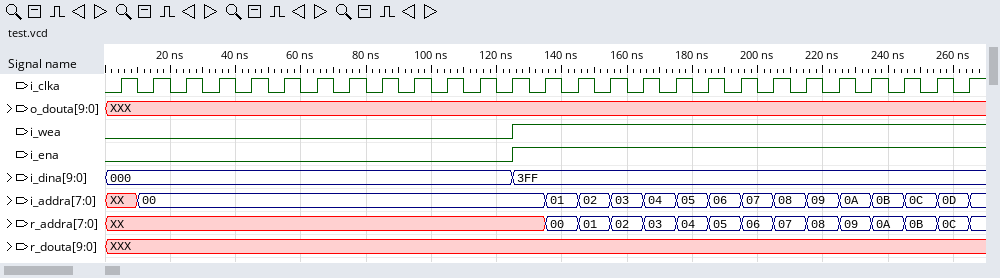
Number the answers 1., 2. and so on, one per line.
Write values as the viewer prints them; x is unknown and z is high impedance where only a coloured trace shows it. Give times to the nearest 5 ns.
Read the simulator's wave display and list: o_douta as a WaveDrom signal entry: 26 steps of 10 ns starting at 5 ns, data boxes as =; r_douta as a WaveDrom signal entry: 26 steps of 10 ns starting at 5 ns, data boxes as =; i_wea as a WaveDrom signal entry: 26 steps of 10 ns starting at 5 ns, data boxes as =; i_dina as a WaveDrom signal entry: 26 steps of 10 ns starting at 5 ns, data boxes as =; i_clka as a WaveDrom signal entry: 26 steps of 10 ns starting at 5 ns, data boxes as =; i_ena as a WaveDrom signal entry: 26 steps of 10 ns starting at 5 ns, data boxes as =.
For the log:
1. {name: 'o_douta', wave: 'x.........................'}
2. {name: 'r_douta', wave: 'x.........................'}
3. {name: 'i_wea', wave: '0...........1.............'}
4. {name: 'i_dina', wave: '=...........=.............', data: '000 3FF'}
5. {name: 'i_clka', wave: 'p.........................'}
6. {name: 'i_ena', wave: '0...........1.............'}
